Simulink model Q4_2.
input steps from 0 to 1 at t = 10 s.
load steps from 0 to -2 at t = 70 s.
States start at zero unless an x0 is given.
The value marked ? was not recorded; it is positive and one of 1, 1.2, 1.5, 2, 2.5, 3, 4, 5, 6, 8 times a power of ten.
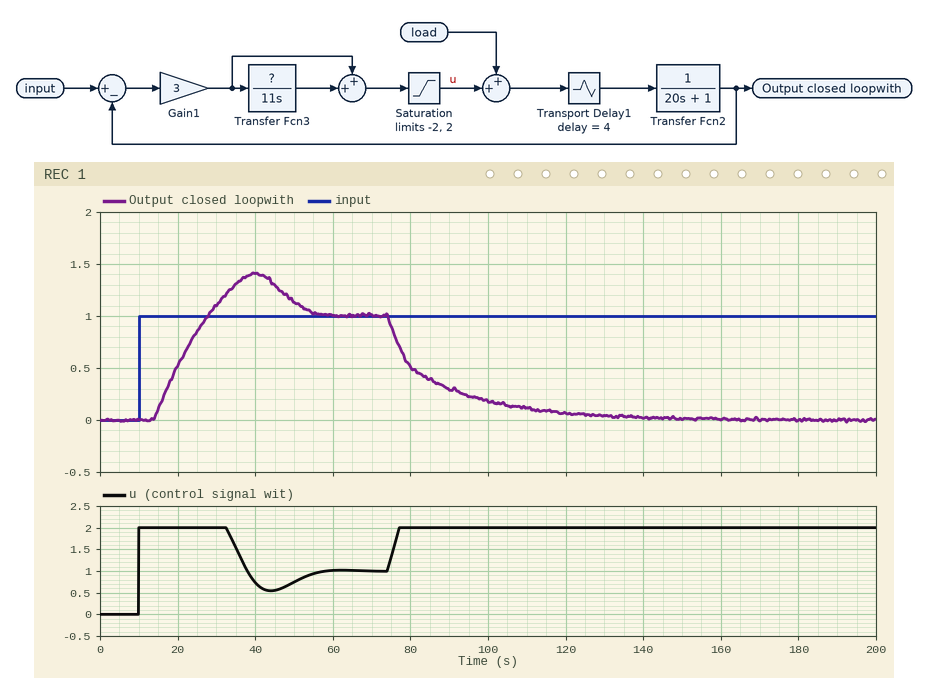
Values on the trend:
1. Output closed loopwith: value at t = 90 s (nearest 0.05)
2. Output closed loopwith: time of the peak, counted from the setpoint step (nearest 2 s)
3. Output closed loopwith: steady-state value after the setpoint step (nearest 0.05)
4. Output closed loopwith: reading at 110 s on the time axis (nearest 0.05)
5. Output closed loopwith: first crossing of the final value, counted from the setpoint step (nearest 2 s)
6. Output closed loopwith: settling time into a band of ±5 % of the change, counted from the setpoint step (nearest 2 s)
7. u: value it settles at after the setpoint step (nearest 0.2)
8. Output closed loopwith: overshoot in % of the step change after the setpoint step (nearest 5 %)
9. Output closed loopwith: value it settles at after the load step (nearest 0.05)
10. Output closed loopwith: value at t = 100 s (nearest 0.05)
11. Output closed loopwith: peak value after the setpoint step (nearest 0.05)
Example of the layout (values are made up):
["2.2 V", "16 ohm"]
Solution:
["0.30", "30 s", "1.00", "0.10", "18 s", "44 s", "1.0", "40 %", "0.00", "0.20", "1.40"]
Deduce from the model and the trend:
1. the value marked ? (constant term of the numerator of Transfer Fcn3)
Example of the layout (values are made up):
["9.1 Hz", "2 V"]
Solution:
["1"]
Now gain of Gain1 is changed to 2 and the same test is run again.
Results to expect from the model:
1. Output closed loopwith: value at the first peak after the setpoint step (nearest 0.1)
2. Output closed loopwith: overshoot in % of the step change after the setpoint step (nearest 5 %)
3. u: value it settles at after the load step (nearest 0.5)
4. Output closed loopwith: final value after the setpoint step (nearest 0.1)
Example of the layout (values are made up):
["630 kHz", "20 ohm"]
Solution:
["1.3", "25 %", "2.0", "1.0"]
